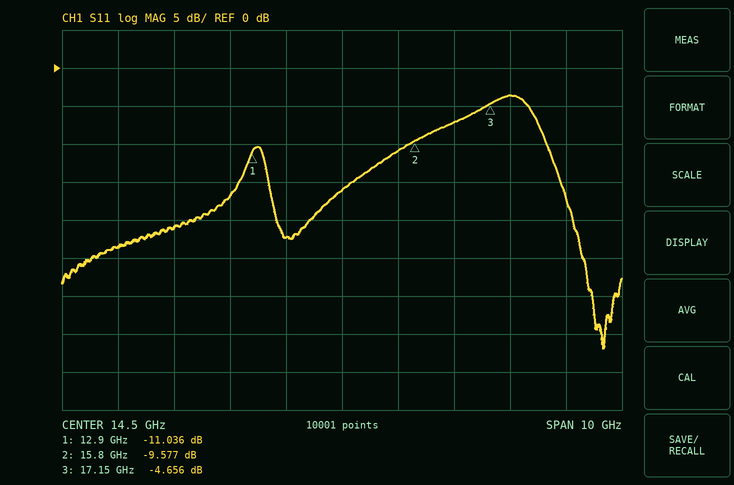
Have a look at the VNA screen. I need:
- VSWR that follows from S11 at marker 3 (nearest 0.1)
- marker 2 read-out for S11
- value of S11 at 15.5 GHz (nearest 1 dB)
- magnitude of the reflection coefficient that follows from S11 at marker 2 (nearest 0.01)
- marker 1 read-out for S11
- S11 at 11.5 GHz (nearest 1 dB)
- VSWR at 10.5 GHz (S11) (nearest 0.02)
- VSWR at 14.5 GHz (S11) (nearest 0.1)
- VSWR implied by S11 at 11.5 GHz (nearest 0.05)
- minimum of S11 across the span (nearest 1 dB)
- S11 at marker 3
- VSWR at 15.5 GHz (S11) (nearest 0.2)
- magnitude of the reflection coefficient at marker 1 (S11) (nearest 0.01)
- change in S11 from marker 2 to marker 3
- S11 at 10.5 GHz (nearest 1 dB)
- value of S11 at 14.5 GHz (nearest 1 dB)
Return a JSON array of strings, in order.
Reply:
["3.8", "-9.577 dB", "-11 dB", "0.33", "-11.036 dB", "-21 dB", "1.14", "1.4", "1.20", "-37 dB", "-4.656 dB", "1.8", "0.28", "4.921 dB", "-24 dB", "-16 dB"]
